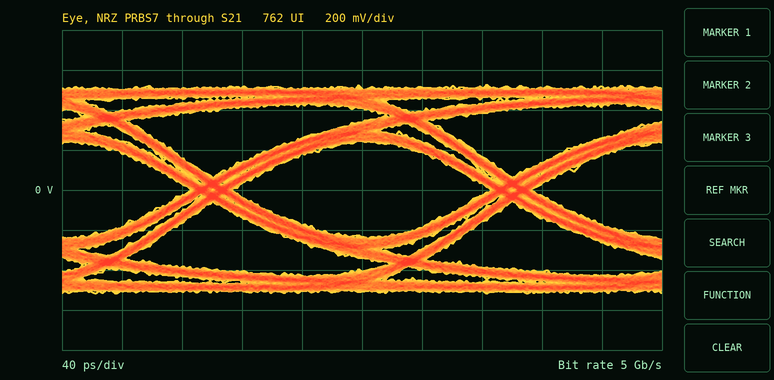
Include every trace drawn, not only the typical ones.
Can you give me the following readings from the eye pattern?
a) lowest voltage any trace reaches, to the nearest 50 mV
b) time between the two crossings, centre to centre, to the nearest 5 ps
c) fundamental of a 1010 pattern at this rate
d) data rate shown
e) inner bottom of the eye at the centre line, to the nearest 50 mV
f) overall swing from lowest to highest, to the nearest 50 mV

-500 mV
200 ps
2.5 GHz
5 Gb/s
-250 mV
1.05 V
